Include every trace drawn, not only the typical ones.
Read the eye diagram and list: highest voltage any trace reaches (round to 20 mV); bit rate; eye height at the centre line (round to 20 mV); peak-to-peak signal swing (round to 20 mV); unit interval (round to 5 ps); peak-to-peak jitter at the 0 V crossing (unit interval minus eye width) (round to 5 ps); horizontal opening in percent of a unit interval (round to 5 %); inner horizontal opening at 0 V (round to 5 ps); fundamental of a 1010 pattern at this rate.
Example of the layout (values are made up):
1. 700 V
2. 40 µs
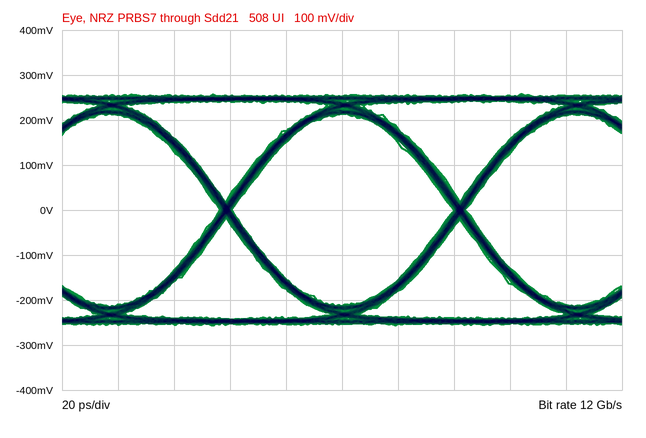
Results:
1. 260 mV
2. 12 Gb/s
3. 420 mV
4. 520 mV
5. 85 ps
6. 5 ps
7. 95 %
8. 80 ps
9. 6 GHz
